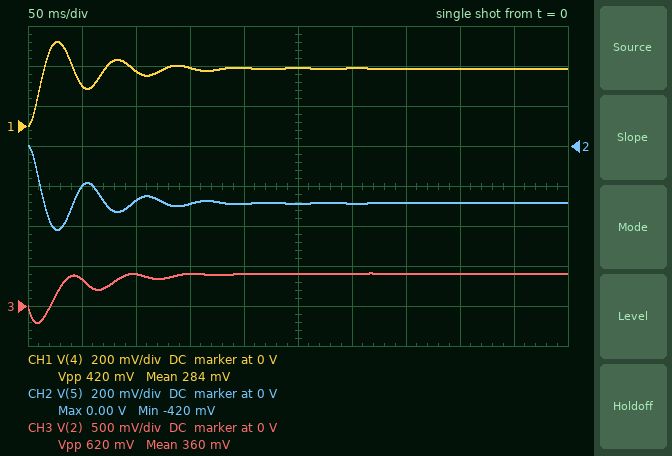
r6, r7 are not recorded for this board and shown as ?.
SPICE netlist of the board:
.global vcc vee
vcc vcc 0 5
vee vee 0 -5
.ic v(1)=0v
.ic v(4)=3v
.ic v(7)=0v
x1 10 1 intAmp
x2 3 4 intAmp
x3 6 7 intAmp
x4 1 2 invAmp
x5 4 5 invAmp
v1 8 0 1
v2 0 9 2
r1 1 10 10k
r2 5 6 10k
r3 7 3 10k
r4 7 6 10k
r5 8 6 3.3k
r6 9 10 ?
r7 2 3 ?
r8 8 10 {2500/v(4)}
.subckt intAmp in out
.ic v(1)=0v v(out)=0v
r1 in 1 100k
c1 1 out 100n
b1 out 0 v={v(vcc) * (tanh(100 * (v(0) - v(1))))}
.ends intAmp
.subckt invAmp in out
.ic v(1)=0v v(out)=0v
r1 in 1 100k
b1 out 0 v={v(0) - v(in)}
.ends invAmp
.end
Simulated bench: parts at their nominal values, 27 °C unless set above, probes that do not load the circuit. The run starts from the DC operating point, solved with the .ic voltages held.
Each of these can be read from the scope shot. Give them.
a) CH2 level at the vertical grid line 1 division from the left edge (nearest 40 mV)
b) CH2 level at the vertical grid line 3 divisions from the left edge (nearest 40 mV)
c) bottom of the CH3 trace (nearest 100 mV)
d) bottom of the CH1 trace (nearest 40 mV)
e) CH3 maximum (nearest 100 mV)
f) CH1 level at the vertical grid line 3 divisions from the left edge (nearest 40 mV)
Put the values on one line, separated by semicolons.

-200 mV; -280 mV; -200 mV; 0 V; 400 mV; 280 mV
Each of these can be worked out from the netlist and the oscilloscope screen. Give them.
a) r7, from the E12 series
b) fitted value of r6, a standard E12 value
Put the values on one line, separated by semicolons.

1.5 kΩ; 27 kΩ
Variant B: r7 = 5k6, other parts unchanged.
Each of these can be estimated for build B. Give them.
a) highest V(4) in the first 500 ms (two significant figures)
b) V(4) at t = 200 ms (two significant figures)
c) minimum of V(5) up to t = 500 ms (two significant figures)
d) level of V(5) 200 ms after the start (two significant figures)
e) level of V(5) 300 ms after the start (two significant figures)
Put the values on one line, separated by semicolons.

770 mV; 550 mV; -770 mV; -550 mV; -530 mV
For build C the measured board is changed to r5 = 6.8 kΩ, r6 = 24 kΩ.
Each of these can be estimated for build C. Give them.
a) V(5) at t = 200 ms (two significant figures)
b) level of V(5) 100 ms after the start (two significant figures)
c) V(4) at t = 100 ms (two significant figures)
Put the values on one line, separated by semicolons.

-260 mV; -240 mV; 240 mV
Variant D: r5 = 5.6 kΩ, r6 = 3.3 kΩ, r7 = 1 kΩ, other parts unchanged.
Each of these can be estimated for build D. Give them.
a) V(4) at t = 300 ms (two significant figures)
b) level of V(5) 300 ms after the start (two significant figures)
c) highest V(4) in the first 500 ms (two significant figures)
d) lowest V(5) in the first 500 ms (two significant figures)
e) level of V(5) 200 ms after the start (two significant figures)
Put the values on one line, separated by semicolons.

1.3 V; -1.3 V; 3.3 V; -3.3 V; -1.0 V
